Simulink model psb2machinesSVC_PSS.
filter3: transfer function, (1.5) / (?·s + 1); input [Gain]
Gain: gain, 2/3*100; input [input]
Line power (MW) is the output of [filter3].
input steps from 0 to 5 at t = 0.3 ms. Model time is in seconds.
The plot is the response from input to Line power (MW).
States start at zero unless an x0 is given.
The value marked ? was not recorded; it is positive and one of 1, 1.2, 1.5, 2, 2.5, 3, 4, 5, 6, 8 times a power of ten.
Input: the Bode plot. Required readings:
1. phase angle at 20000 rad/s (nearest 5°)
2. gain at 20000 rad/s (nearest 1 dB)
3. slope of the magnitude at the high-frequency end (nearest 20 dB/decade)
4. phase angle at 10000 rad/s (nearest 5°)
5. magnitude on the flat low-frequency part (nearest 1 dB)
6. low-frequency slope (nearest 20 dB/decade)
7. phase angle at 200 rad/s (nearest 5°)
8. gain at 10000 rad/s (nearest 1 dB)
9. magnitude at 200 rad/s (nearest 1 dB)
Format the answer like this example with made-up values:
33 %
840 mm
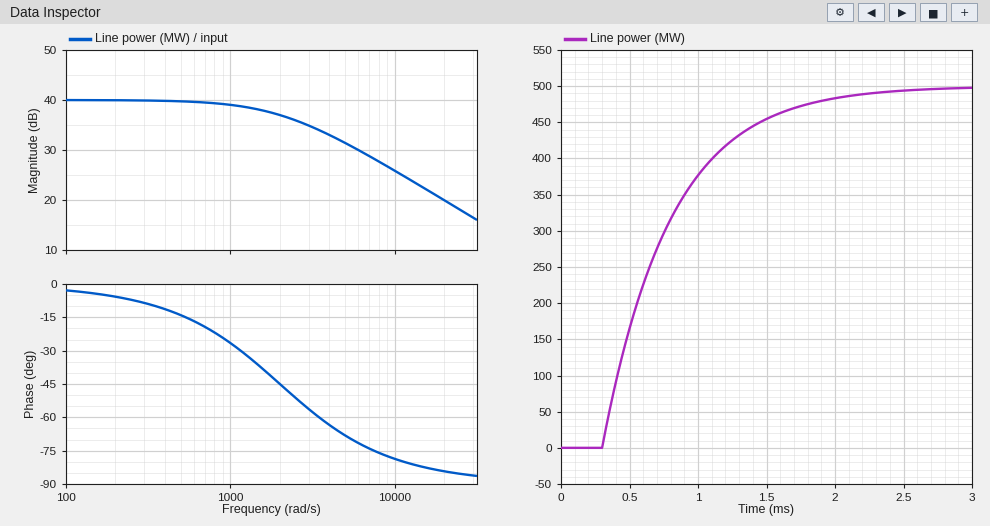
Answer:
-85°
20 dB
-20 dB/decade
-80°
40 dB
0 dB/decade
-5°
26 dB
40 dB
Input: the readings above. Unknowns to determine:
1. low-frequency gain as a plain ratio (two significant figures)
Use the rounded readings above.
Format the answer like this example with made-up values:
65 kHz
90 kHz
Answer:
100
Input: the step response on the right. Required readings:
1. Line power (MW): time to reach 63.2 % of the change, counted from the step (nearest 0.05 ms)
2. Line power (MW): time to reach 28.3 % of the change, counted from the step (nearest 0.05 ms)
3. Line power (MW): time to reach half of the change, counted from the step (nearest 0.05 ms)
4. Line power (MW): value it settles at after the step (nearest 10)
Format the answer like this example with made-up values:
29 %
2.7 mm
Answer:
0.50 ms
0.15 ms
0.35 ms
500
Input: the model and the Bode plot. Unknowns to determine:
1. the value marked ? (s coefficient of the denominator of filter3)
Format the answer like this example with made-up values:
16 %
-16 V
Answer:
0.0005
